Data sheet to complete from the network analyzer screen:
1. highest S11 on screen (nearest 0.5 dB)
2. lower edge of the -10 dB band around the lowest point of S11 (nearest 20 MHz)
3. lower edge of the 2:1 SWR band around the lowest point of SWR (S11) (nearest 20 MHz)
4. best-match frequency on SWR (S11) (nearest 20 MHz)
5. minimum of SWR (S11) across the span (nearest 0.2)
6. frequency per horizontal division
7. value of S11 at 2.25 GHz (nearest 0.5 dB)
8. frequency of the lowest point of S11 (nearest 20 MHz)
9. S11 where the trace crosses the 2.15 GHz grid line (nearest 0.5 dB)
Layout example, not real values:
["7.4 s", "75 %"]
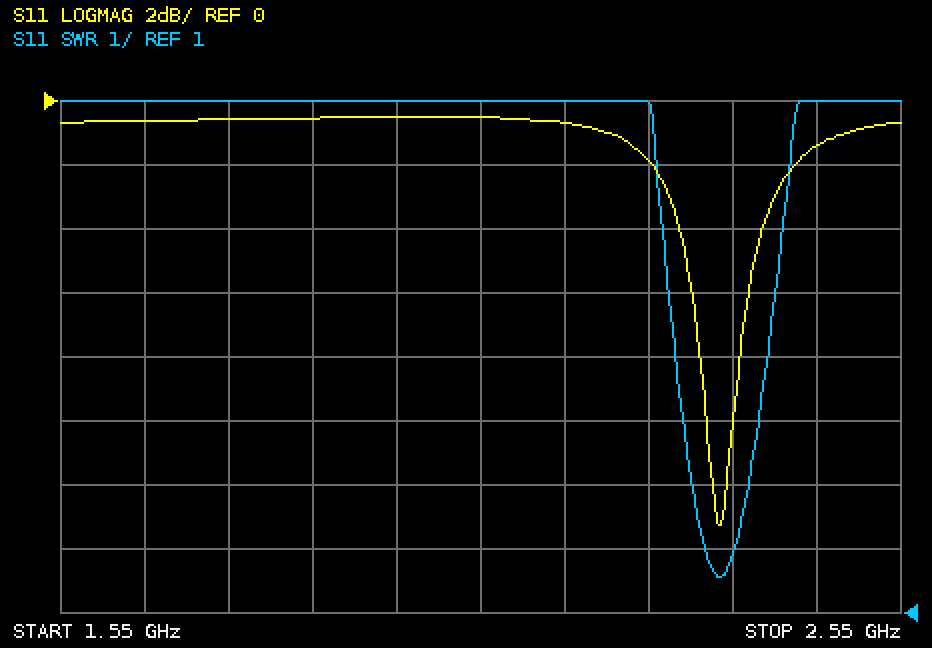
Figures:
["-0.5 dB", "2.32 GHz", "2.32 GHz", "2.34 GHz", "1.6", "100 MHz", "-2.0 dB", "2.34 GHz", "-0.5 dB"]
